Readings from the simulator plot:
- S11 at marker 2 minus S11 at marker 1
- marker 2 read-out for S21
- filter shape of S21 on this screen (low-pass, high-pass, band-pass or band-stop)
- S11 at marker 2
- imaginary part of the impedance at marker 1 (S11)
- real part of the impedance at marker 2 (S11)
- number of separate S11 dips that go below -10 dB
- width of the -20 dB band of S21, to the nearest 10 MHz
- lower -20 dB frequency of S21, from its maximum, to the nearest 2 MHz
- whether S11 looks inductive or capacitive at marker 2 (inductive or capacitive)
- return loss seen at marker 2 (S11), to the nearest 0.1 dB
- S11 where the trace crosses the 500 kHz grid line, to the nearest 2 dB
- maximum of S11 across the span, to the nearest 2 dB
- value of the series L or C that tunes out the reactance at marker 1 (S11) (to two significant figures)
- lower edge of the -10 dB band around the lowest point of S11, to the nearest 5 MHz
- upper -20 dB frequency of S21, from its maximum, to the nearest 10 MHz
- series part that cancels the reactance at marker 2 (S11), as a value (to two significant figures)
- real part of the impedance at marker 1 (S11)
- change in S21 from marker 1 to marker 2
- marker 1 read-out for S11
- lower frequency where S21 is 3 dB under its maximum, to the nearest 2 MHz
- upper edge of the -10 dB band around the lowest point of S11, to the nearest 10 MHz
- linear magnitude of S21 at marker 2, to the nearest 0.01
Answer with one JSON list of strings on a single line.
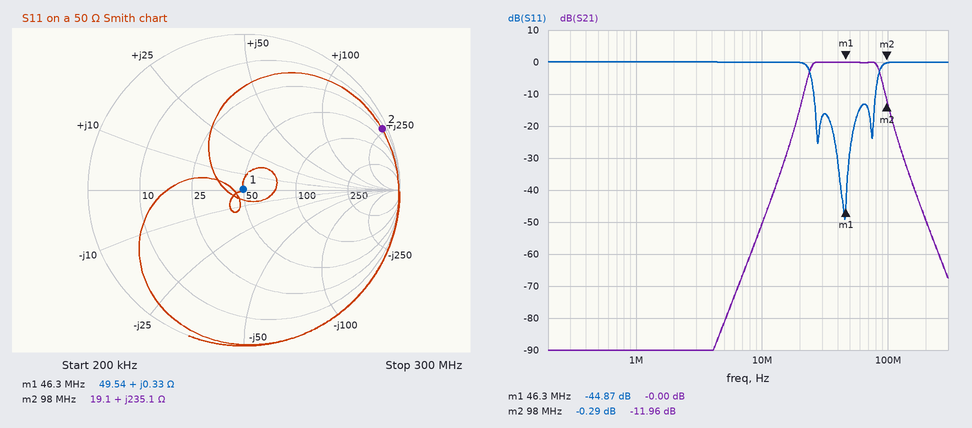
["44.58 dB", "-11.96 dB", "band-pass", "-0.29 dB", "+0.33 Ω", "19.1 Ω", "3", "90 MHz", "18 MHz", "inductive", "0.3 dB", "0 dB", "0 dB", "10 nF", "25 MHz", "110 MHz", "6.9 pF", "49.54 Ω", "-11.96 dB", "-44.87 dB", "24 MHz", "80 MHz", "0.25"]
